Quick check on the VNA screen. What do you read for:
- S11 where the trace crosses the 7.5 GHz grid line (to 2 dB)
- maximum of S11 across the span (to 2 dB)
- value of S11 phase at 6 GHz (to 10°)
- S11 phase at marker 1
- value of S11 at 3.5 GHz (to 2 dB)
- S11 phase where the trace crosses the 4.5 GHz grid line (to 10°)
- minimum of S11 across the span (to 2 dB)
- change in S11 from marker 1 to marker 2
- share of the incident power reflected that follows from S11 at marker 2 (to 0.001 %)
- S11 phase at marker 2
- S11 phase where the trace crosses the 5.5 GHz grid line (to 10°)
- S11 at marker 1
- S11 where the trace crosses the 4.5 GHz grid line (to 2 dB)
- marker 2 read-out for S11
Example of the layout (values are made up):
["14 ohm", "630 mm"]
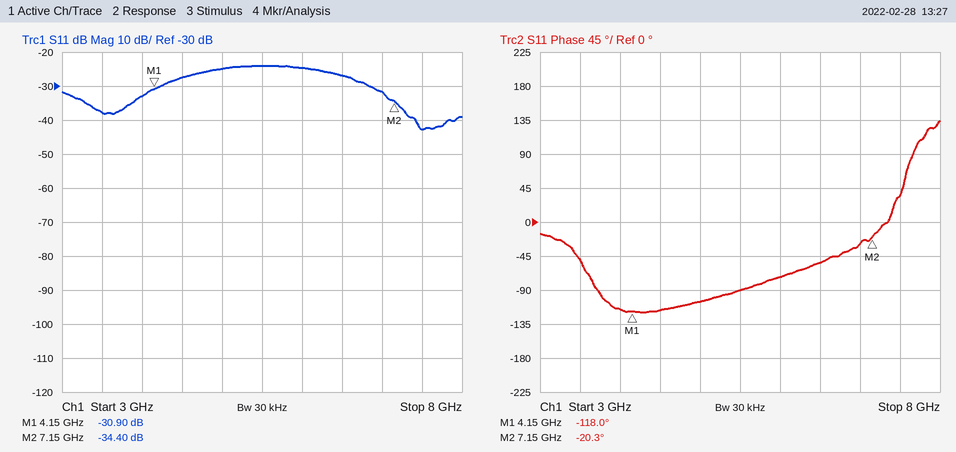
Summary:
["-42 dB", "-24 dB", "-70°", "-118.0°", "-38 dB", "-120°", "-42 dB", "-3.50 dB", "0.036 %", "-20.3°", "-90°", "-30.90 dB", "-28 dB", "-34.40 dB"]
